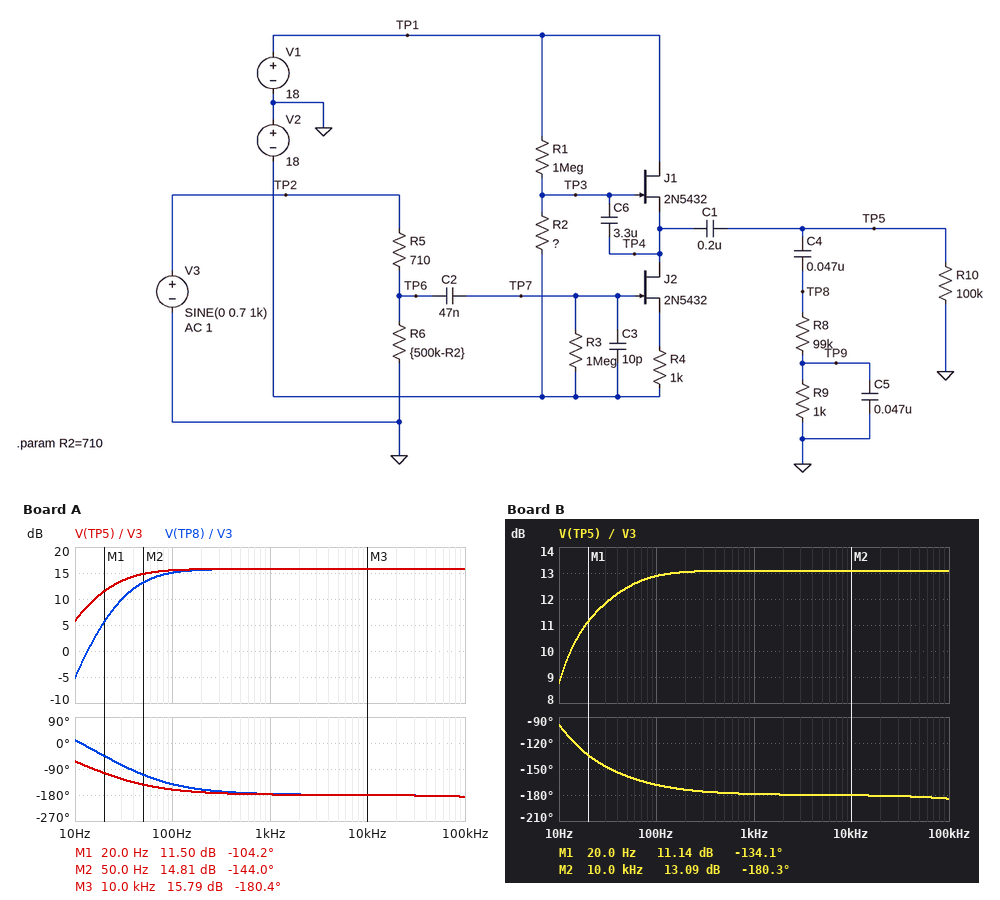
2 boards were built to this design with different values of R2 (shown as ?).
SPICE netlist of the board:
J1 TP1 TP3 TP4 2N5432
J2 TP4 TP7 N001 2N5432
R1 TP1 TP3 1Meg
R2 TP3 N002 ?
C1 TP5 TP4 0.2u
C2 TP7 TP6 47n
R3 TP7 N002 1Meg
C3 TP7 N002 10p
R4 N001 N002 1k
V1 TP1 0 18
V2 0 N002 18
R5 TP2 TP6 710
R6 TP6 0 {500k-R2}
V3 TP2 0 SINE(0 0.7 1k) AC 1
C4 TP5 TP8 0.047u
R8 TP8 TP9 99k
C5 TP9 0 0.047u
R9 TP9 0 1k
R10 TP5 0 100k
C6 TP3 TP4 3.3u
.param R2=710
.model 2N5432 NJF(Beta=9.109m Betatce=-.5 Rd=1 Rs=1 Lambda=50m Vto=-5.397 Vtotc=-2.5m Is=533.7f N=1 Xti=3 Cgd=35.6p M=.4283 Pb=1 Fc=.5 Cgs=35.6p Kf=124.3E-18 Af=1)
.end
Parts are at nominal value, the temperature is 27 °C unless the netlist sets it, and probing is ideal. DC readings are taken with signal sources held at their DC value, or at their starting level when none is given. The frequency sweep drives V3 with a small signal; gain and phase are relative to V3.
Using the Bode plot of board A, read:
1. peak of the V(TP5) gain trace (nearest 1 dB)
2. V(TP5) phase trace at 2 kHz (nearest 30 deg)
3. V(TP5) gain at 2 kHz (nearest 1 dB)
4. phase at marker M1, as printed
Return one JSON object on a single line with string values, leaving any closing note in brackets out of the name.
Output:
{"peak of the V(TP5) gain trace": "16 dB", "V(TP5) phase trace at 2 kHz": "-180 deg", "V(TP5) gain at 2 kHz": "16 dB", "phase at marker M1, as printed": "-104.2 deg"}
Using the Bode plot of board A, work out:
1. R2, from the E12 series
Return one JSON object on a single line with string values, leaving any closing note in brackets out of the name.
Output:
{"R2, from the E12 series": "470 kΩ"}
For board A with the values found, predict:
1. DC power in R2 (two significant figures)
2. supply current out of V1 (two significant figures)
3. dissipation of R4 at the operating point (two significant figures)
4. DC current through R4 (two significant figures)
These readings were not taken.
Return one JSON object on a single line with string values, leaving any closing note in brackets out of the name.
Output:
{"DC power in R2": "280 µW", "supply current out of V1": "4.8 mA", "dissipation of R4 at the operating point": "23 mW", "DC current through R4": "4.8 mA"}
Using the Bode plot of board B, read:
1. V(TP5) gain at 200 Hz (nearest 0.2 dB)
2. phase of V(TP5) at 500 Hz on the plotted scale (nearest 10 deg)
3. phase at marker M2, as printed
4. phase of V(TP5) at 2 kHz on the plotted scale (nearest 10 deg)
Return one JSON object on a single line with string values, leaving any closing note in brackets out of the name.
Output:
{"V(TP5) gain at 200 Hz": "13.0 dB", "phase of V(TP5) at 500 Hz on the plotted scale": "-180 deg", "phase at marker M2, as printed": "-180.3 deg", "phase of V(TP5) at 2 kHz on the plotted scale": "-180 deg"}
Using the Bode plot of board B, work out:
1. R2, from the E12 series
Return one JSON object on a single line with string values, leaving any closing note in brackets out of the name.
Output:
{"R2, from the E12 series": "2.2 MΩ"}
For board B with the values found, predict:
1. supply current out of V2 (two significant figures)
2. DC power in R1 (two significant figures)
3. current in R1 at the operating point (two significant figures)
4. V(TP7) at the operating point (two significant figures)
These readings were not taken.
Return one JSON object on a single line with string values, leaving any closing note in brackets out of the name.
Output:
{"supply current out of V2": "4.9 mA", "DC power in R1": "130 µW", "current in R1 at the operating point": "11 µA", "V(TP7) at the operating point": "-18 V"}
